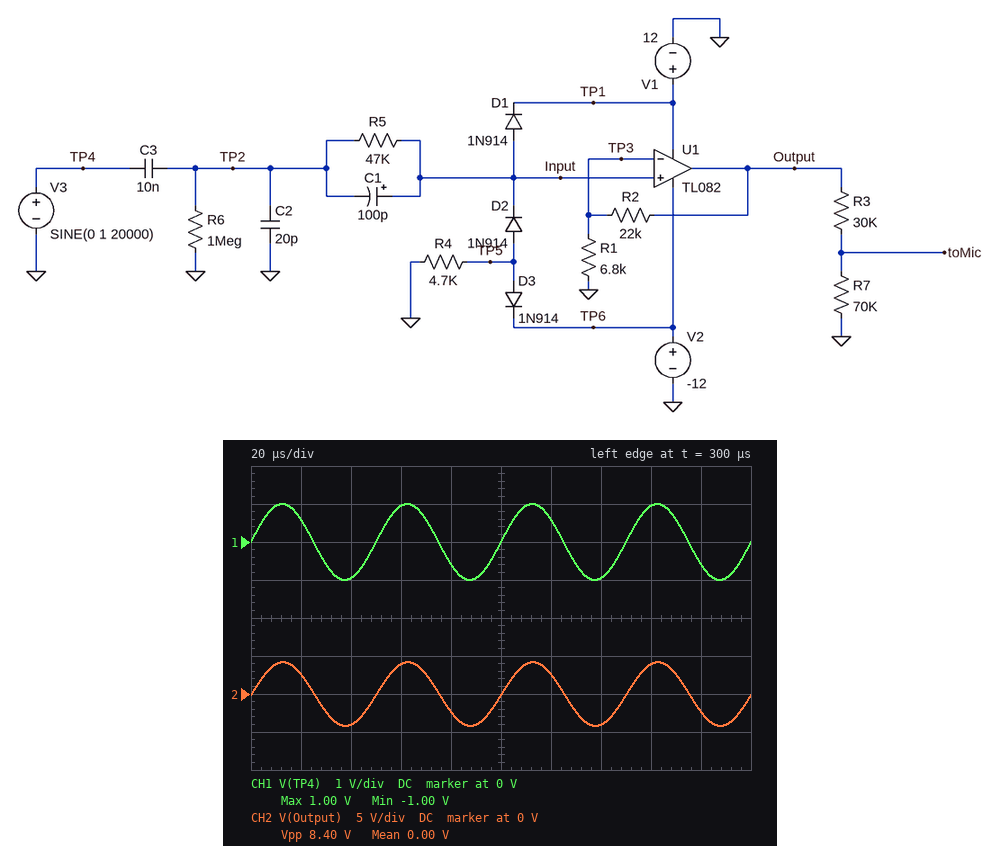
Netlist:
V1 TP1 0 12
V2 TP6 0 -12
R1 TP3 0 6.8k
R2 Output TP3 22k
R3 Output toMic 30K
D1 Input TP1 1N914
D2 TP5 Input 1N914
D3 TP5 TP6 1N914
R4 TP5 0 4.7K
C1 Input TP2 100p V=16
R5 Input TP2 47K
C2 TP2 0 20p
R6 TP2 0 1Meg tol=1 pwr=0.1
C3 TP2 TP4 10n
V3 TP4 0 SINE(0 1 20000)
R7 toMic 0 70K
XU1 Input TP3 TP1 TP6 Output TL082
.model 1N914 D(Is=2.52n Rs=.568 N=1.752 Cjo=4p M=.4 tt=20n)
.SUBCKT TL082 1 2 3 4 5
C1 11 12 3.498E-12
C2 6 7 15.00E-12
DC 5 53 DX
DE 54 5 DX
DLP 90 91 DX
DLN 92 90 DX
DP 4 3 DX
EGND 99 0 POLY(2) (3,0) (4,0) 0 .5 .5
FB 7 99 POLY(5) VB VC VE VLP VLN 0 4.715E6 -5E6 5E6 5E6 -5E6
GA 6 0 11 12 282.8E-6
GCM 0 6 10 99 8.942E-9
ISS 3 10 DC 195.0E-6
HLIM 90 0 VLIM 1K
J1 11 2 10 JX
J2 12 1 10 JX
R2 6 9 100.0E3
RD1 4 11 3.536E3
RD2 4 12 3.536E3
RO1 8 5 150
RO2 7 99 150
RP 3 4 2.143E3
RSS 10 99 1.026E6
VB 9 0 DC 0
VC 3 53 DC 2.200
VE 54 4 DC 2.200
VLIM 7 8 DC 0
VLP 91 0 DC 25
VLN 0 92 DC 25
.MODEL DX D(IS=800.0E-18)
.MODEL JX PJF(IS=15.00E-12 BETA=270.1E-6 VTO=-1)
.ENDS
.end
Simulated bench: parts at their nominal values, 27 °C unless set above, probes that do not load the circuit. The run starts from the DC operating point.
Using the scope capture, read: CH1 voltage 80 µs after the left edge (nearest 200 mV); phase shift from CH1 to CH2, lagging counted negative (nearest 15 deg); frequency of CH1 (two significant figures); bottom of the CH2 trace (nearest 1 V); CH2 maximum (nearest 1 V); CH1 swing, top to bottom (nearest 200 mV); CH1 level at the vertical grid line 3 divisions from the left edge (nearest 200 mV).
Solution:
-600 mV
0 deg
20 kHz
-4 V
4 V
2.0 V
1.0 V
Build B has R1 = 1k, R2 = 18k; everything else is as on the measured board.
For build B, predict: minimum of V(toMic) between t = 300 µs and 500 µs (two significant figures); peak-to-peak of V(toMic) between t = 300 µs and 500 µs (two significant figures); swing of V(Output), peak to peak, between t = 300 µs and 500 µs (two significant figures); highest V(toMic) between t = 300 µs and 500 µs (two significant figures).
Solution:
-7.3 V
15 V
21 V
7.3 V
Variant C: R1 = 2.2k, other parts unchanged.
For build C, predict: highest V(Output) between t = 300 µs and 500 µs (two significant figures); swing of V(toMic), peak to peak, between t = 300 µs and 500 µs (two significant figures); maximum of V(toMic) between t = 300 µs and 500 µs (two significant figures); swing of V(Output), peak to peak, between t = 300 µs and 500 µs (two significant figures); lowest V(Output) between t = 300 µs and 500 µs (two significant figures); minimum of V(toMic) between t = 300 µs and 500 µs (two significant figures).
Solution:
10 V
15 V
7.3 V
21 V
-10 V
-7.3 V
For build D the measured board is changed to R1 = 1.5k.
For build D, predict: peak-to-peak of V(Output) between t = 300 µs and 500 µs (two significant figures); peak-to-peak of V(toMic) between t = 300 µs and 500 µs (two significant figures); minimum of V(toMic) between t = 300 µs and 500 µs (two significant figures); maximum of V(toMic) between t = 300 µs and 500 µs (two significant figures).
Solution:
21 V
15 V
-7.3 V
7.3 V
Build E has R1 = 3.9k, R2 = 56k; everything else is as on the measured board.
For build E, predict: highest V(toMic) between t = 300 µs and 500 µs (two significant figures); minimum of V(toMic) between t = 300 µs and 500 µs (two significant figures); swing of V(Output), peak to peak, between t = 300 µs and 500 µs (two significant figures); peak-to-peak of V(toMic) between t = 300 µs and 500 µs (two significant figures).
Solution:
7.3 V
-7.3 V
21 V
15 V
